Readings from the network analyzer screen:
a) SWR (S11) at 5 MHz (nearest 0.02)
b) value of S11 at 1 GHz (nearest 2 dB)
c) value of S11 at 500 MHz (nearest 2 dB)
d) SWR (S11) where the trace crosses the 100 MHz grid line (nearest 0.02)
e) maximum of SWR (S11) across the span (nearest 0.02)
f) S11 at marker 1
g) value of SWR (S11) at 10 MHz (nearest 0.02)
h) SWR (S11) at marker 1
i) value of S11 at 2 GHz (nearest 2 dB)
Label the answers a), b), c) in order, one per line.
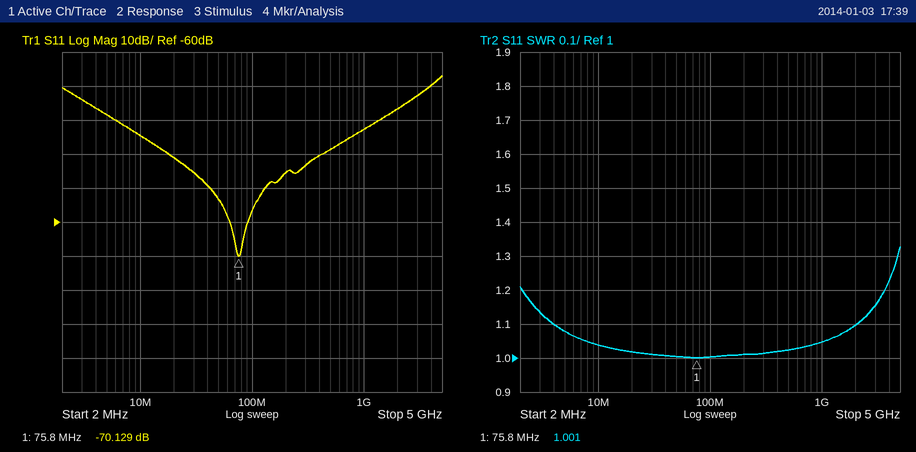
a) 1.08
b) -32 dB
c) -38 dB
d) 1.00
e) 1.32
f) -70.129 dB
g) 1.04
h) 1.001
i) -26 dB
